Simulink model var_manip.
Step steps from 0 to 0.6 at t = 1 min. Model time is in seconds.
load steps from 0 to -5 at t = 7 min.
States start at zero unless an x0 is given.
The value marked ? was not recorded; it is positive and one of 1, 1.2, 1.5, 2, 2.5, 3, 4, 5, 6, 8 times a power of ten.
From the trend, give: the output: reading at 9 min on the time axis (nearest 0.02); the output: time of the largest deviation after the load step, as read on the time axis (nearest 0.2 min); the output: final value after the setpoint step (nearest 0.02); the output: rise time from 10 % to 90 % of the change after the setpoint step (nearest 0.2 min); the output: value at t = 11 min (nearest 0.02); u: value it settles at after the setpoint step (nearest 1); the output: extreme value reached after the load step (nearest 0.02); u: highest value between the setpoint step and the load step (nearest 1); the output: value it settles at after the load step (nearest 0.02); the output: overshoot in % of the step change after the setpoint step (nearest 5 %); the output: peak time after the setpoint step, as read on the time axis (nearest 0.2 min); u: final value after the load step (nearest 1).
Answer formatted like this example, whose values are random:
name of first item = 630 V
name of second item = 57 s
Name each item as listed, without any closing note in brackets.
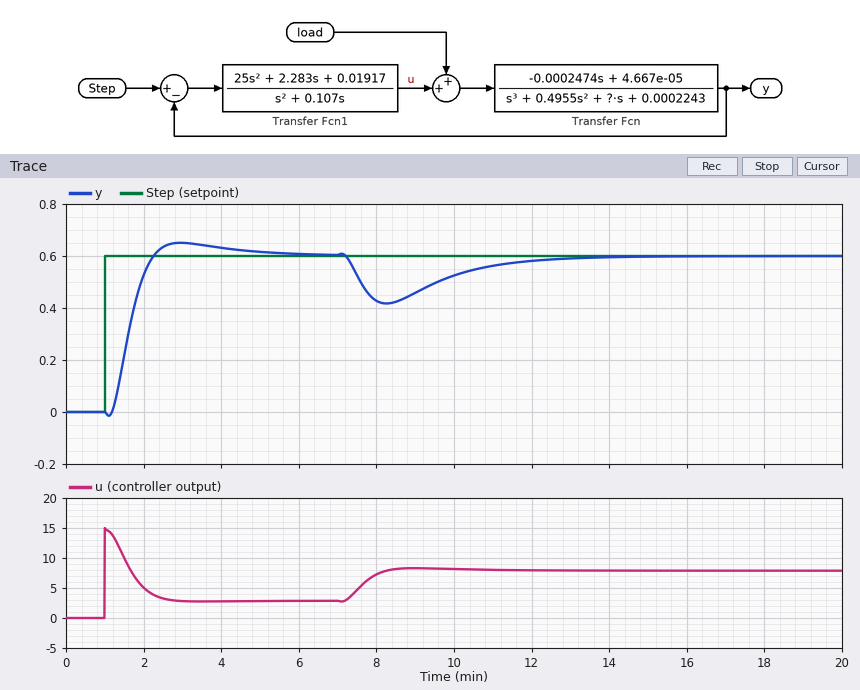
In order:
the output: reading at 9 min on the time axis = 0.46
the output: time of the largest deviation after the load step, as read on the time axis = 8.2 min
the output: final value after the setpoint step = 0.60
the output: rise time from 10 % to 90 % of the change after the setpoint step = 0.8 min
the output: value at t = 11 min = 0.56
u: value it settles at after the setpoint step = 3
the output: extreme value reached after the load step = 0.42
u: highest value between the setpoint step and the load step = 15
the output: value it settles at after the load step = 0.60
the output: overshoot in % of the step change after the setpoint step = 10 %
the output: peak time after the setpoint step, as read on the time axis = 3.0 min
u: final value after the load step = 8
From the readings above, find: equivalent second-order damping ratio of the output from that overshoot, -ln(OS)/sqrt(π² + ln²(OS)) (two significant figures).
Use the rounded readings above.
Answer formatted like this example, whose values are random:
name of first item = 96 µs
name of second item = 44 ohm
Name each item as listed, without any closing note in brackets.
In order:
equivalent second-order damping ratio of the output from that overshoot, -ln(OS)/sqrt(π² + ln²(OS)) = 0.59
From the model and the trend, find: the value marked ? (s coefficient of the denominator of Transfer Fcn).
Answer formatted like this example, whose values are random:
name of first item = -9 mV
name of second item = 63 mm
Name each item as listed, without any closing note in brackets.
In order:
the value marked ? = 0.04
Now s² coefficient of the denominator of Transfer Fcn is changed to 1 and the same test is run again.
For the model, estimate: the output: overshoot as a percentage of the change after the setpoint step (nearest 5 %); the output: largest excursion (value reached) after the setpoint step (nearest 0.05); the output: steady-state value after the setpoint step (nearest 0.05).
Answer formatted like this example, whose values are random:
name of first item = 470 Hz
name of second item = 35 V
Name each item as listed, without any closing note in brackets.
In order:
the output: overshoot as a percentage of the change after the setpoint step = 25 %
the output: largest excursion (value reached) after the setpoint step = 0.75
the output: steady-state value after the setpoint step = 0.60
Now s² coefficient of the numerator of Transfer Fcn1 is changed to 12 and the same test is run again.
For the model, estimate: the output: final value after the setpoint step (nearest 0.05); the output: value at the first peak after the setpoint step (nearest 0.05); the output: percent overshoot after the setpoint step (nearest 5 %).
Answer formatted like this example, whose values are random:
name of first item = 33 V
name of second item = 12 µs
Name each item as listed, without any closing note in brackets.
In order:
the output: final value after the setpoint step = 0.60
the output: value at the first peak after the setpoint step = 0.70
the output: percent overshoot after the setpoint step = 15 %
